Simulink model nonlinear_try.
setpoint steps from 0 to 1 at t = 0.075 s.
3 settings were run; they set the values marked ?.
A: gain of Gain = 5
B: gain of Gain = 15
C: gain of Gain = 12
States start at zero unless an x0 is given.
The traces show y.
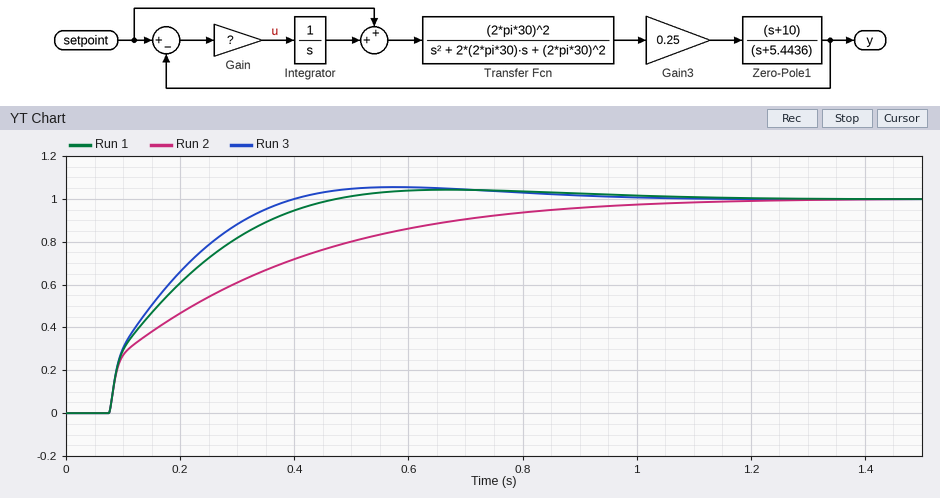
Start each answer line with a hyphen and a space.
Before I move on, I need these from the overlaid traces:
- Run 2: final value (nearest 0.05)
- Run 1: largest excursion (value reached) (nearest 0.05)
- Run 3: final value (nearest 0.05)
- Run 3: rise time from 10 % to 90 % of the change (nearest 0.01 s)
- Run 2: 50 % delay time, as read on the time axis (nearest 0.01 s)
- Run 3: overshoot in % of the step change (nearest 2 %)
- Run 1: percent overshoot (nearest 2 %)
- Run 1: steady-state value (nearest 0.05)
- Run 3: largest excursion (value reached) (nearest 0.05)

- 1.00
- 1.05
- 1.00
- 0.23 s
- 0.22 s
- 6 %
- 4 %
- 1.00
- 1.05
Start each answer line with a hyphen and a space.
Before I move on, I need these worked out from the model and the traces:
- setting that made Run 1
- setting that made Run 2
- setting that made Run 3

- C
- A
- B
